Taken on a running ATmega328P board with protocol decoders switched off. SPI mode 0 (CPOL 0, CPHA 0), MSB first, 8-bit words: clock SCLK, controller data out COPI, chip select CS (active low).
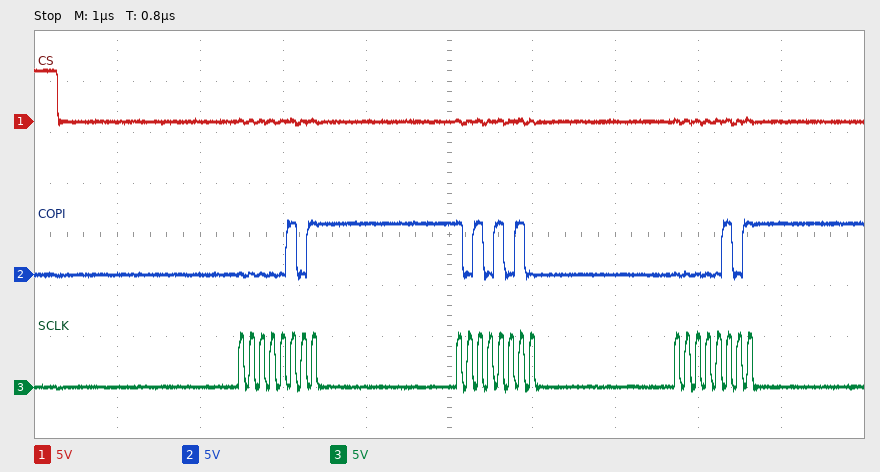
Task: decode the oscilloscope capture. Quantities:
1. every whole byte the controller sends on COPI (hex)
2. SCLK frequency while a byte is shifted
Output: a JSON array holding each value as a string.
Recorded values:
["05 AA 05", "8 MHz"]
